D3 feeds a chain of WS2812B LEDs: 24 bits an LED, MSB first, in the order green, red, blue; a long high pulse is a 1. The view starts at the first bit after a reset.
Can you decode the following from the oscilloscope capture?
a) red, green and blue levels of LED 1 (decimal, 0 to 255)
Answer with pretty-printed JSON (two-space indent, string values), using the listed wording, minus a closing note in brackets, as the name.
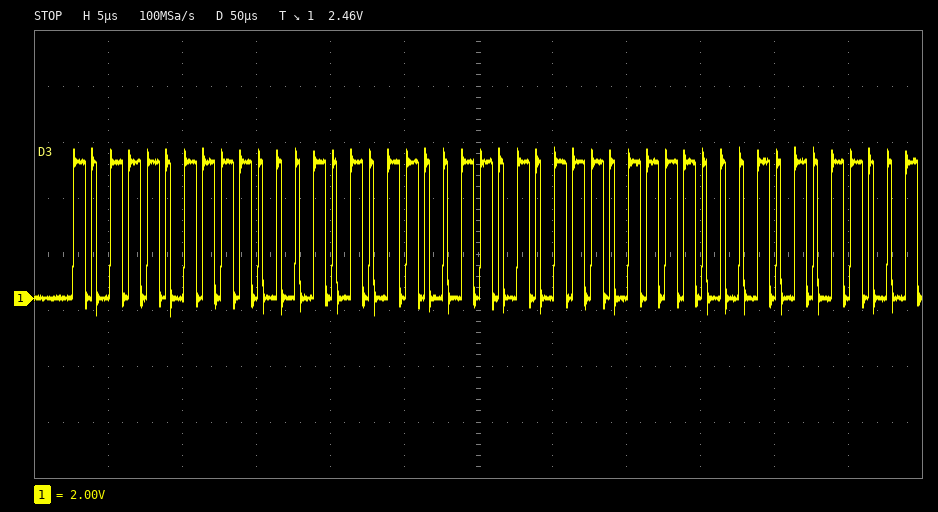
{
  "red, green and blue levels of LED 1": "197, 187, 102"
}
